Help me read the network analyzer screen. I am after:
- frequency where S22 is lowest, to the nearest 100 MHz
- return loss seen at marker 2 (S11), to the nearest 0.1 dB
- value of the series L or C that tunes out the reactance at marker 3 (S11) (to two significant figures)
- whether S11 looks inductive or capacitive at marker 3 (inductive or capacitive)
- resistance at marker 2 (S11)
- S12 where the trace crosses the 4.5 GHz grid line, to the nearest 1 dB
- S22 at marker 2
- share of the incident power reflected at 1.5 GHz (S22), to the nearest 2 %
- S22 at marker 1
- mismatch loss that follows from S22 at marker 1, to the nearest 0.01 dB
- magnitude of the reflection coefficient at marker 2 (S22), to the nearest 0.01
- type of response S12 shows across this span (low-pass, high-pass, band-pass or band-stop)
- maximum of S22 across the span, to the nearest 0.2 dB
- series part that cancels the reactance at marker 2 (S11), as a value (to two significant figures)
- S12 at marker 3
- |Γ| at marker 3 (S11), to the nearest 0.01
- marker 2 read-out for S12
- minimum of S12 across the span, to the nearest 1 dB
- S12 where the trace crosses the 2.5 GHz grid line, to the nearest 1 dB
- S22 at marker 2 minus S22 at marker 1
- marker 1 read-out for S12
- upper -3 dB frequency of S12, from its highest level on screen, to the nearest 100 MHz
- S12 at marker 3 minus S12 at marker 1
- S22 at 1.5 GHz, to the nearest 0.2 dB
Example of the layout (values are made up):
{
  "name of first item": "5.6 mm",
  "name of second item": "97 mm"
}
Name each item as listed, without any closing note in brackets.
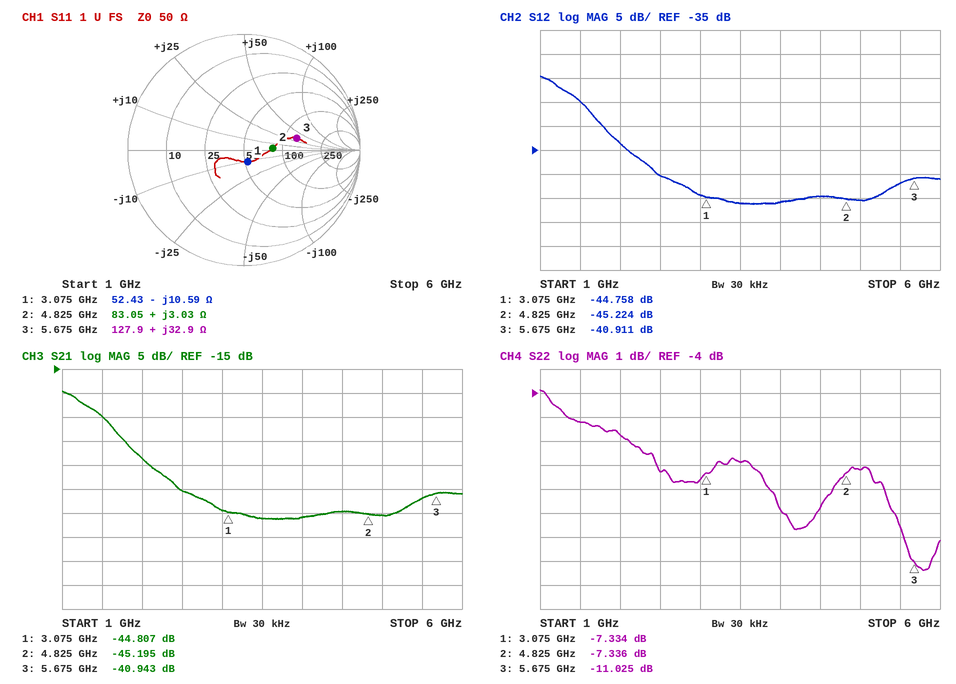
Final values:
{
  "frequency where S22 is lowest, to the nearest 100 MHz": "5.8 GHz",
  "return loss seen at marker 2 (S11), to the nearest 0.1 dB": "12.1 dB",
  "value of the series L or C that tunes out the reactance at marker 3 (S11)": "850 fF",
  "whether S11 looks inductive or capacitive at marker 3": "inductive",
  "resistance at marker 2": "83.05 Ω",
  "S12 where the trace crosses the 4.5 GHz grid line, to the nearest 1 dB": "-45 dB",
  "S22 at marker 2": "-7.336 dB",
  "share of the incident power reflected at 1.5 GHz (S22), to the nearest 2 %": "30 %",
  "S22 at marker 1": "-7.334 dB",
  "mismatch loss that follows from S22 at marker 1, to the nearest 0.01 dB": "0.89 dB",
  "magnitude of the reflection coefficient at marker 2 (S22), to the nearest 0.01": "0.43",
  "type of response S12 shows across this span": "low-pass",
  "maximum of S22 across the span, to the nearest 0.2 dB": "-3.8 dB",
  "series part that cancels the reactance at marker 2 (S11), as a value": "11 pF",
  "S12 at marker 3": "-40.911 dB",
  "|Γ| at marker 3 (S11), to the nearest 0.01": "0.47",
  "marker 2 read-out for S12": "-45.224 dB",
  "minimum of S12 across the span, to the nearest 1 dB": "-46 dB",
  "S12 where the trace crosses the 2.5 GHz grid line, to the nearest 1 dB": "-40 dB",
  "S22 at marker 2 minus S22 at marker 1": "-0.002 dB",
  "marker 1 read-out for S12": "-44.758 dB",
  "upper -3 dB frequency of S12, from its highest level on screen, to the nearest 100 MHz": "1.3 GHz",
  "S12 at marker 3 minus S12 at marker 1": "3.847 dB",
  "S22 at 1.5 GHz, to the nearest 0.2 dB": "-5.2 dB"
}
